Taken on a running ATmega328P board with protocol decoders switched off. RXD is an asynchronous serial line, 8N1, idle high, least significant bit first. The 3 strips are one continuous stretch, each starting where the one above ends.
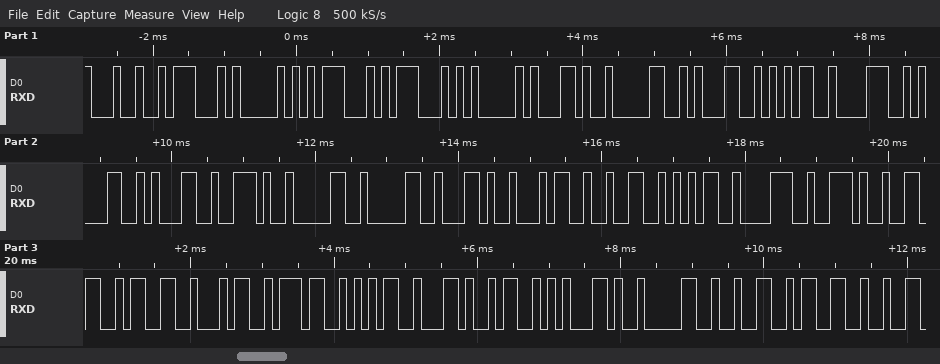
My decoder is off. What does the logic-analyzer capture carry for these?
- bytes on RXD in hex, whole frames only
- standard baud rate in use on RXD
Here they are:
24 47 50 47 47 41 2C 30 31 35 38 31 31 2E 30 30 2C 34 32 35 38 2E 36 33 34 37 35 2C 53 2C 30 32 33
9600 baud
